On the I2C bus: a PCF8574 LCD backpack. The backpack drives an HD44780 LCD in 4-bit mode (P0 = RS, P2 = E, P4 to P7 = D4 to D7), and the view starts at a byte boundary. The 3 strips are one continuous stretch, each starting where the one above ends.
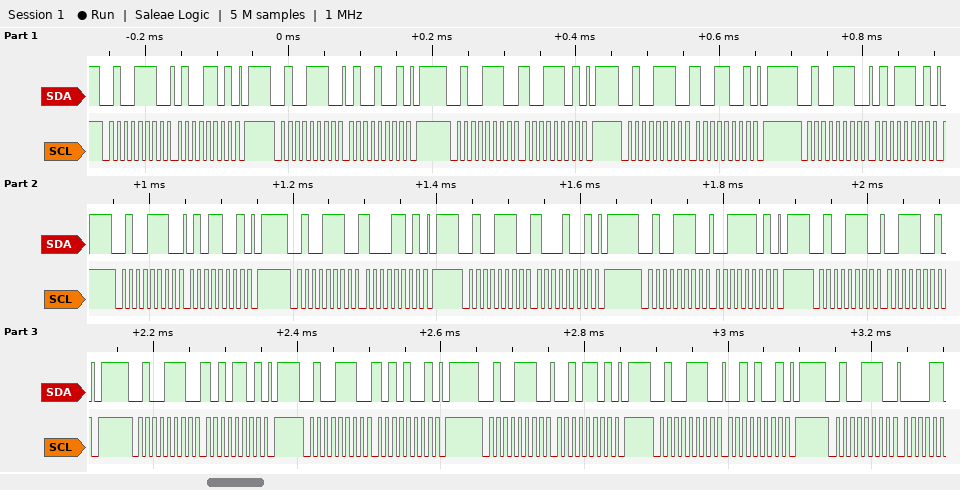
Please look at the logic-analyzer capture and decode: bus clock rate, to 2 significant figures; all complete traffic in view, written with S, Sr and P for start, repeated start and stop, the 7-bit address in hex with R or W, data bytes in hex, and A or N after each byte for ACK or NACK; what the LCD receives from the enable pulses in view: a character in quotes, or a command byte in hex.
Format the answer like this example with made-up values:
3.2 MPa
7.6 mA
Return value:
100 kHz
S 27W A 4D A P S 27W A 49 A P S 27W A 9D A P S 27W A 99 A P S 27W A 5D A P S 27W A 59 A P S 27W A 8D A P S 27W A 89 A P S 27W A 3D A P S 27W A 39 A P S 27W A AD A P S 27W A A9 A P S 27W A 2D A P S 27W A 29 A P S 27W A
'I' 'X' ':'
